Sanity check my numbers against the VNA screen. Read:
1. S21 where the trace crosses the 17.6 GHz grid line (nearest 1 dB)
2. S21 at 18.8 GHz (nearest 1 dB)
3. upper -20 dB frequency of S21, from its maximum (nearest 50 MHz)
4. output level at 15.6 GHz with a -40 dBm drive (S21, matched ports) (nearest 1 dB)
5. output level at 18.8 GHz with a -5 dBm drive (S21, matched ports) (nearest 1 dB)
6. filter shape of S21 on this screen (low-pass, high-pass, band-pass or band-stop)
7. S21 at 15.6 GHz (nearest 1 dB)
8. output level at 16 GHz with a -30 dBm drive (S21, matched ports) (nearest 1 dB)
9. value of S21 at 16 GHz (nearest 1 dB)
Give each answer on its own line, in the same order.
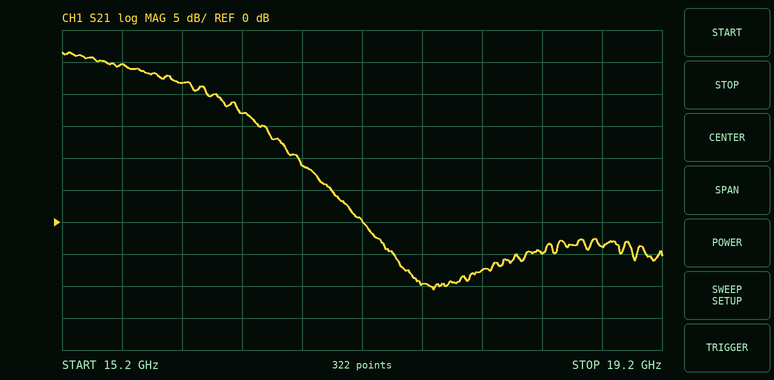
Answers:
-10 dB
-4 dB
16.90 GHz
-15 dBm
-9 dBm
low-pass
25 dB
-8 dBm
22 dB
